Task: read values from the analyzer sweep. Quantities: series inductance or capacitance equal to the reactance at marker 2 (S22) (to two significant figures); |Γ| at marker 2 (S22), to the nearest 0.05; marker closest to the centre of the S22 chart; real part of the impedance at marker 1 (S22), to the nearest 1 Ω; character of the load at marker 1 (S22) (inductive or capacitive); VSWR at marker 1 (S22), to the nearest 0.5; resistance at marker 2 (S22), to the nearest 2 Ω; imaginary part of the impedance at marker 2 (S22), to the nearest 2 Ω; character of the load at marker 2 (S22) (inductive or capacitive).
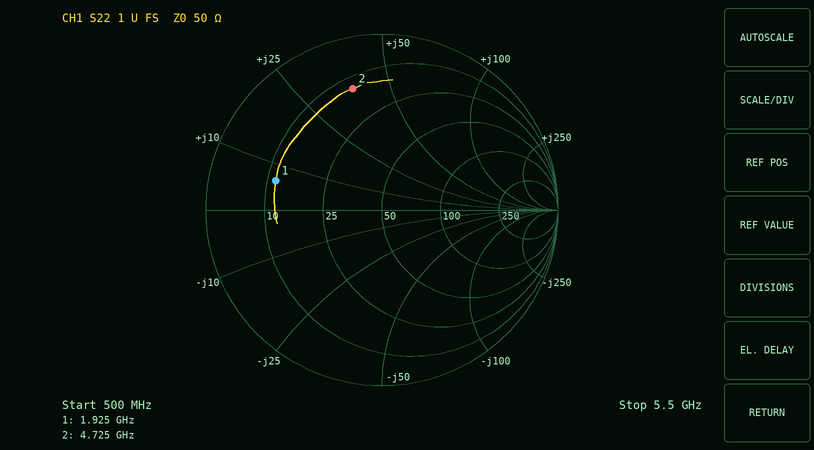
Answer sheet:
1.3 nH
0.70
marker 1
12 Ω
inductive
4.5
14 Ω
+38 Ω
inductive
